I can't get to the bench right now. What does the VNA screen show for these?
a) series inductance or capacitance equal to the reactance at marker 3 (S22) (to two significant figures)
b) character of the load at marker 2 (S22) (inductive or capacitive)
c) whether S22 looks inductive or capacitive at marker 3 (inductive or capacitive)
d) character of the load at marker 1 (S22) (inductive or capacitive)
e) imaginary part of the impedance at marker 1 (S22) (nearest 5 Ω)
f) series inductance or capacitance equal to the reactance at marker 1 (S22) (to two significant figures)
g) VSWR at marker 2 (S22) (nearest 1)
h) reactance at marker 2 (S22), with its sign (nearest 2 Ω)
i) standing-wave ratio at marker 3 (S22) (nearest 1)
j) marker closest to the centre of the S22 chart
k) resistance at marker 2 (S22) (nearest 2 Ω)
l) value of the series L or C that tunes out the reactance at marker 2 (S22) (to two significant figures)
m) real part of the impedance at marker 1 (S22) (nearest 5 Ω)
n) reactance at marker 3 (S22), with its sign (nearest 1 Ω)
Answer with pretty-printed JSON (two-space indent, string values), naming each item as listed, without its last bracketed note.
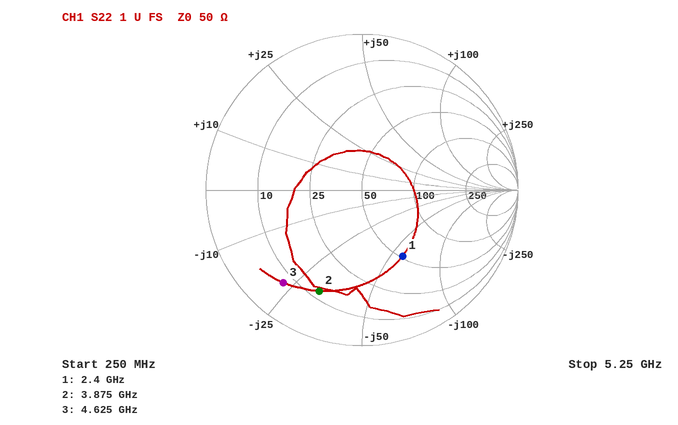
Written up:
{
  "series inductance or capacitance equal to the reactance at marker 3 (S22)": "1.5 pF",
  "character of the load at marker 2 (S22)": "capacitive",
  "whether S22 looks inductive or capacitive at marker 3": "capacitive",
  "character of the load at marker 1 (S22)": "capacitive",
  "imaginary part of the impedance at marker 1 (S22)": "-60 Ω",
  "series inductance or capacitance equal to the reactance at marker 1 (S22)": "1.1 pF",
  "VSWR at marker 2 (S22)": "6",
  "reactance at marker 2 (S22), with its sign": "-32 Ω",
  "standing-wave ratio at marker 3 (S22)": "8",
  "marker closest to the centre of the S22 chart": "marker 1",
  "resistance at marker 2 (S22)": "12 Ω",
  "value of the series L or C that tunes out the reactance at marker 2 (S22)": "1.3 nH",
  "real part of the impedance at marker 1 (S22)": "50 Ω",
  "reactance at marker 3 (S22), with its sign": "-23 Ω"
}
